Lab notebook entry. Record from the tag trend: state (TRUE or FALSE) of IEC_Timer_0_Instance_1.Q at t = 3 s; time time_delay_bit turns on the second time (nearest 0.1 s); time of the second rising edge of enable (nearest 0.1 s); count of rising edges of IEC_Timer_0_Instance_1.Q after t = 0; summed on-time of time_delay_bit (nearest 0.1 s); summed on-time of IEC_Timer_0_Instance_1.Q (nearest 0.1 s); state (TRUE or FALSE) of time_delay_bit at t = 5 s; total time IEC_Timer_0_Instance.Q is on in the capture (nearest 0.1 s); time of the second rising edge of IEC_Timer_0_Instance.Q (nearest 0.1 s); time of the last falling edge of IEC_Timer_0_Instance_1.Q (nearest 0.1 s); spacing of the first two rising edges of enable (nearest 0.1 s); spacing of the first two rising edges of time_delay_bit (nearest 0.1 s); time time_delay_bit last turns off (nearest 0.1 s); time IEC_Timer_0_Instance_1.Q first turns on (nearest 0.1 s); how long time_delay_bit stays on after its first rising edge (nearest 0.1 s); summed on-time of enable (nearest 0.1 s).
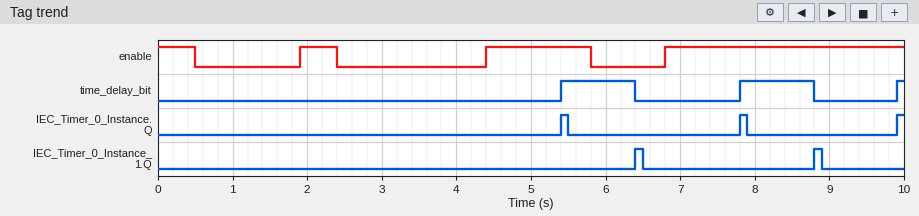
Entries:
FALSE
7.8 s
4.4 s
2
2.1 s
0.2 s
FALSE
0.3 s
7.8 s
8.9 s
2.5 s
2.4 s
8.8 s
6.4 s
1.0 s
5.6 s
